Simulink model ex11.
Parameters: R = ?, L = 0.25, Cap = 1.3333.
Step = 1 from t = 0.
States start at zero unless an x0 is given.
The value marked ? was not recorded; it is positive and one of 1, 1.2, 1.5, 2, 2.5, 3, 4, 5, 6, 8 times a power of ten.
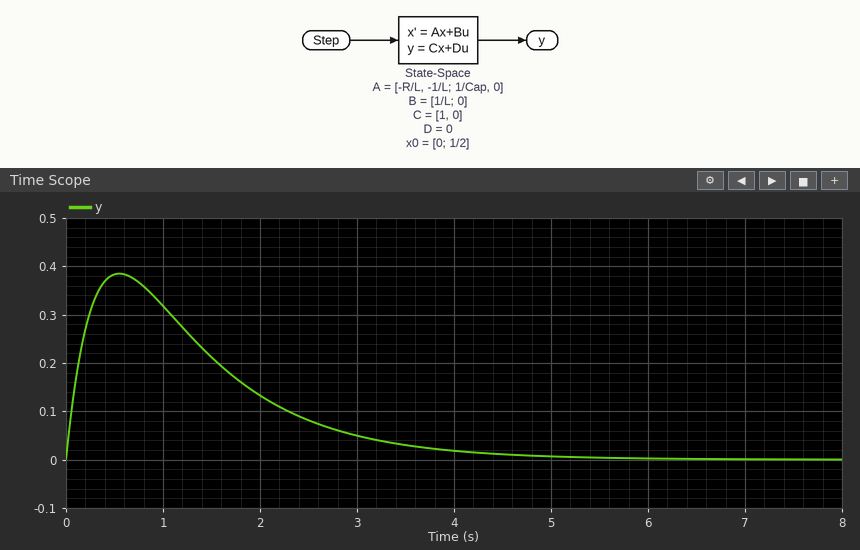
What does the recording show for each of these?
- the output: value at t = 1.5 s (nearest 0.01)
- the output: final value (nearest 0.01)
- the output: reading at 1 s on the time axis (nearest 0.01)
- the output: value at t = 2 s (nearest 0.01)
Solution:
0.21
0.00
0.32
0.13
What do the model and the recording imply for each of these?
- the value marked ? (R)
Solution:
1
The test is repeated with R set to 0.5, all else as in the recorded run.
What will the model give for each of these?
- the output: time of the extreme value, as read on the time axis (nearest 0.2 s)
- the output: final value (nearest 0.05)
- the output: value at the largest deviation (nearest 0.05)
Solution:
0.6 s
0.00
0.60
